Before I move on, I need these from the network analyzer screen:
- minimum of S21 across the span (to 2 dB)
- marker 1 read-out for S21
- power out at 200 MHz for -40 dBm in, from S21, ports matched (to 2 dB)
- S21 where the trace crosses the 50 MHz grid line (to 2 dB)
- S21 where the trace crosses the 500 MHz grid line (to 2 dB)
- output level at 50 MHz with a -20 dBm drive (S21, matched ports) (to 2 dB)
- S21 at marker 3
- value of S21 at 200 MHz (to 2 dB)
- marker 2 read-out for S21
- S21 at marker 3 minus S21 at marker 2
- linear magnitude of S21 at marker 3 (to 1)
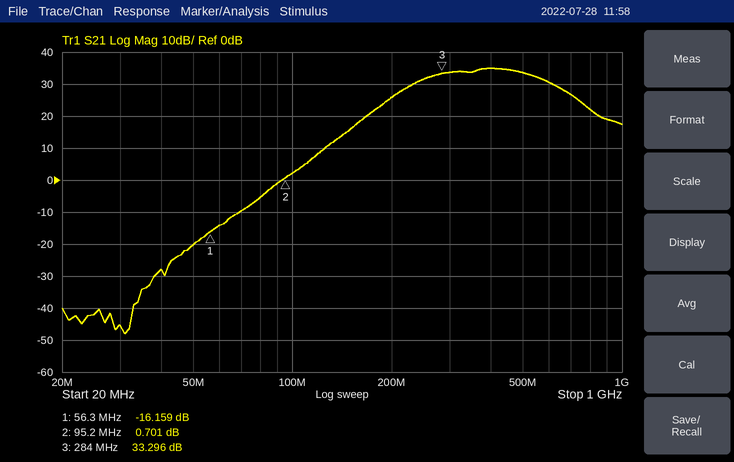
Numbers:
-48 dB
-16.159 dB
-14 dBm
-20 dB
34 dB
-40 dBm
33.296 dB
26 dB
0.701 dB
32.595 dB
46
